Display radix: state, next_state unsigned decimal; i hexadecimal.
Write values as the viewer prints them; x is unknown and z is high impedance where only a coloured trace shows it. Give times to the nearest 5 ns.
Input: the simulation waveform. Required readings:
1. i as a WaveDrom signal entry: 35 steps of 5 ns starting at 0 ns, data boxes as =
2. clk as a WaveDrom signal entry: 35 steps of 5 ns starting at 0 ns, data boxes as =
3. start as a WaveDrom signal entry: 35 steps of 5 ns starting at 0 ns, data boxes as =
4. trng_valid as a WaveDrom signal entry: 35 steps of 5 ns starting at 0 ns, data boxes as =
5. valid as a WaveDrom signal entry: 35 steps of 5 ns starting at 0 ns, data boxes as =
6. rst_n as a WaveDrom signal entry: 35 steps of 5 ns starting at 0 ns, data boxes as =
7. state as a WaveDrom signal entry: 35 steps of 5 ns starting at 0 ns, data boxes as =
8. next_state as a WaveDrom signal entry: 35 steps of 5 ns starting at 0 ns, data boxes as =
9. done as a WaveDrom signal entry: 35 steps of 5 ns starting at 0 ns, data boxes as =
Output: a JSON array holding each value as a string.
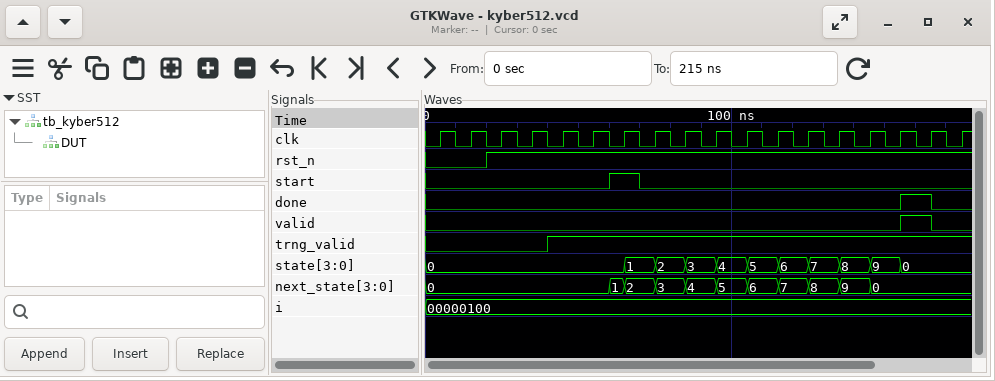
["{name: 'i', wave: '=..................................', data: '00000100'}", "{name: 'clk', wave: '01010101010101010101010101010101010'}", "{name: 'start', wave: '0...........1.0....................'}", "{name: 'trng_valid', wave: '0.......1..........................'}", "{name: 'valid', wave: '0..............................1.0.'}", "{name: 'rst_n', wave: '0...1..............................'}", "{name: 'state', wave: '=............=.=.=.=.=.=.=.=.=.=...', data: '0 1 2 3 4 5 6 7 8 9 0'}", "{name: 'next_state', wave: '=...........==.=.=.=.=.=.=.=.=.....', data: '0 1 2 3 4 5 6 7 8 9 0'}", "{name: 'done', wave: '0..............................1.0.'}"]
